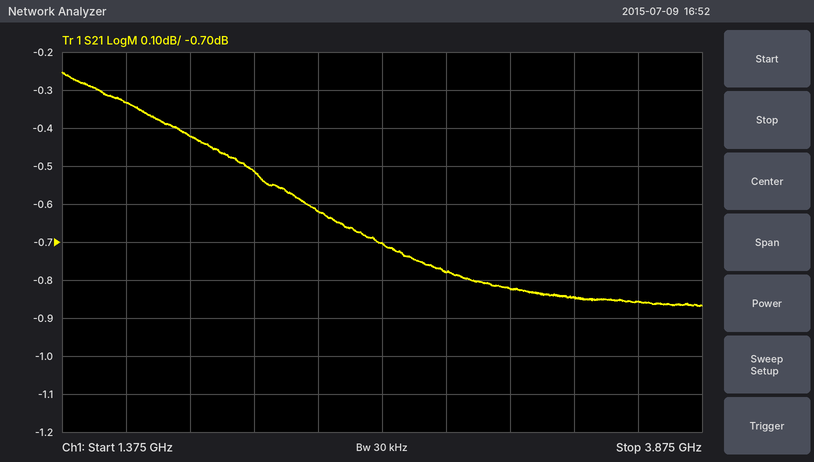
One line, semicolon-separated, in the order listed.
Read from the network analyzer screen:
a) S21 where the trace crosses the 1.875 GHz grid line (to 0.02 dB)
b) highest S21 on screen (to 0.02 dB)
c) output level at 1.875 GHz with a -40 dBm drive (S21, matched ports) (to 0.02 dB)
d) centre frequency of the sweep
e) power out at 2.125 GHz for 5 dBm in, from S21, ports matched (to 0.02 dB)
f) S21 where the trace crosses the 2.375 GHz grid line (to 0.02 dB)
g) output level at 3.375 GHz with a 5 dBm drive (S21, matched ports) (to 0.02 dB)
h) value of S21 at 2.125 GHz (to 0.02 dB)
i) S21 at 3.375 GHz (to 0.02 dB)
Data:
-0.42 dB; -0.26 dB; -40.42 dBm; 2.625 GHz; 4.48 dBm; -0.62 dB; 4.16 dBm; -0.52 dB; -0.84 dB
